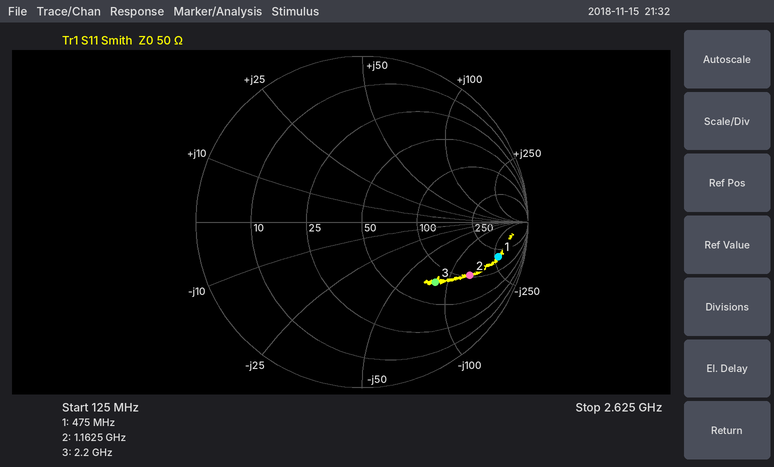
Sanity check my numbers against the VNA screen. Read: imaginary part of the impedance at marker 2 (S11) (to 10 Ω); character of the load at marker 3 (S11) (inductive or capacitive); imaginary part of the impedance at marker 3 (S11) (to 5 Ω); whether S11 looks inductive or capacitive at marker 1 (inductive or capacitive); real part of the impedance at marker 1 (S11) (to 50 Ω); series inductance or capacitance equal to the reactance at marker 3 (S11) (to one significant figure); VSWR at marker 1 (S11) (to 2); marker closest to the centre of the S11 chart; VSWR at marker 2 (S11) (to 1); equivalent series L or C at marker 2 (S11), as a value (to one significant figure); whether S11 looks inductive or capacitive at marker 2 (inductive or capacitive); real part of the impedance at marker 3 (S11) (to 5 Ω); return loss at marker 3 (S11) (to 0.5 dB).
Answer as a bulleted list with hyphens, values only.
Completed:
- -140 Ω
- capacitive
- -80 Ω
- capacitive
- 200 Ω
- 900 fF
- 12
- marker 3
- 6
- 1.0 pF
- capacitive
- 75 Ω
- 5.0 dB
